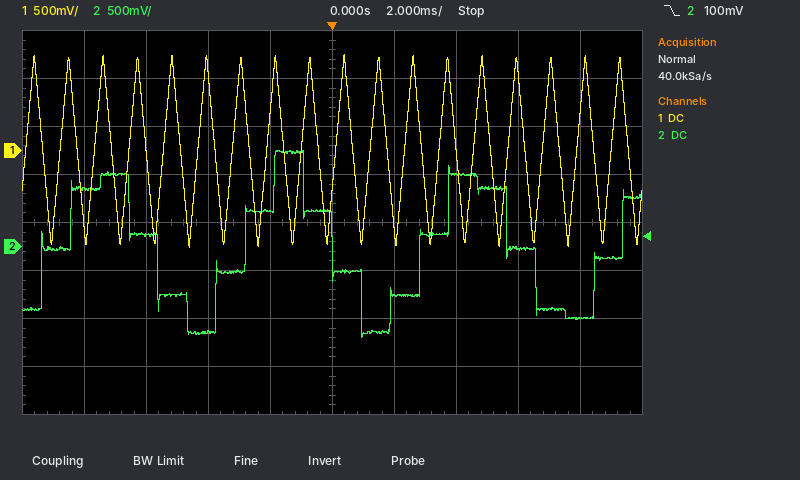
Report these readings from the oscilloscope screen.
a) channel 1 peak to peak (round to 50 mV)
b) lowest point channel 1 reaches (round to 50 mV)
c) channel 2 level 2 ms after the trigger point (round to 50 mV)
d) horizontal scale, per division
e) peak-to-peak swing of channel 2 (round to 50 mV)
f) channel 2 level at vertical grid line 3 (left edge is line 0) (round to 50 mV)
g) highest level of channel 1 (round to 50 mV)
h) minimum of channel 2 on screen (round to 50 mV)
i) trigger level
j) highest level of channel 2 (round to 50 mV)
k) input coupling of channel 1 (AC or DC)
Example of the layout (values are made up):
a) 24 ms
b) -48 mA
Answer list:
a) 2.00 V
b) -1.00 V
c) -500 mV
d) 2 ms
e) 1.95 V
f) -900 mV
g) 1.00 V
h) -950 mV
i) 100 mV
j) 1.00 V
k) DC
